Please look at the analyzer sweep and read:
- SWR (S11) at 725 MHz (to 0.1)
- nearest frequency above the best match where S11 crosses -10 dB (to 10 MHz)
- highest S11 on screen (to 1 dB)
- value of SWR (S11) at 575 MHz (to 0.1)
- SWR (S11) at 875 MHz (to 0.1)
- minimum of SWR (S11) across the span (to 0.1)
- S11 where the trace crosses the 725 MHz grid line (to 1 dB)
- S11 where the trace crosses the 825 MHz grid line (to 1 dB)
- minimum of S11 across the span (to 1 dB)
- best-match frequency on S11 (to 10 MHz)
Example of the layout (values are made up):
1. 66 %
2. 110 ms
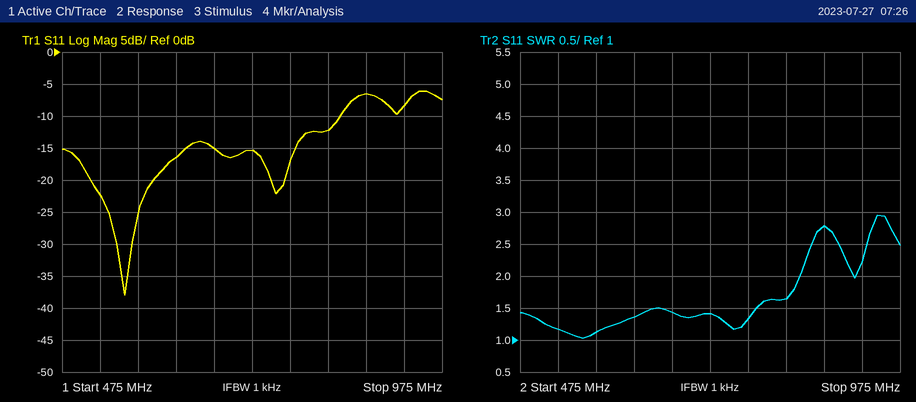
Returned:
1. 1.4
2. 840 MHz
3. -6 dB
4. 1.1
5. 2.8
6. 1.0
7. -15 dB
8. -12 dB
9. -38 dB
10. 560 MHz
